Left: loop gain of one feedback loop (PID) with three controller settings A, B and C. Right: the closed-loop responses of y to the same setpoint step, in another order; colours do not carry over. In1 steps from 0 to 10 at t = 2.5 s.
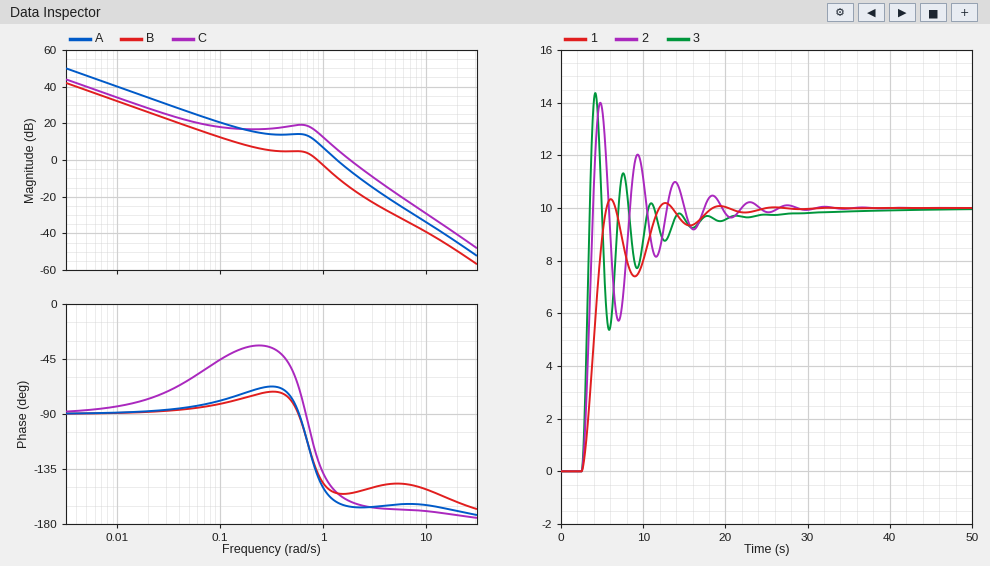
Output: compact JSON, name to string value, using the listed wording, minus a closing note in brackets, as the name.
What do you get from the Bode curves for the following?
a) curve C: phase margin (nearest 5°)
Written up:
{"curve C: phase margin": "20°"}
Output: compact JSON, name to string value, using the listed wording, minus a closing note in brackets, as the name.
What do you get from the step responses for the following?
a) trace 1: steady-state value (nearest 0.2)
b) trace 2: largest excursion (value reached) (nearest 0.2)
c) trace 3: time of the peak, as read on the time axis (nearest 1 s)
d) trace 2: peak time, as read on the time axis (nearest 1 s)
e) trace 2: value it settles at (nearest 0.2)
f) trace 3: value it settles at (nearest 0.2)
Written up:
{"trace 1: steady-state value": "10.0", "trace 2: largest excursion (value reached)": "14.0", "trace 3: time of the peak, as read on the time axis": "4 s", "trace 2: peak time, as read on the time axis": "5 s", "trace 2: value it settles at": "10.0", "trace 3: value it settles at": "10.0"}
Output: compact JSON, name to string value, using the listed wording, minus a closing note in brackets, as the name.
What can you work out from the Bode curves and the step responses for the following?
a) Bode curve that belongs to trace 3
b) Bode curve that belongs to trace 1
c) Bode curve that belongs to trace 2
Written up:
{"Bode curve that belongs to trace 3": "C", "Bode curve that belongs to trace 1": "B", "Bode curve that belongs to trace 2": "A"}
